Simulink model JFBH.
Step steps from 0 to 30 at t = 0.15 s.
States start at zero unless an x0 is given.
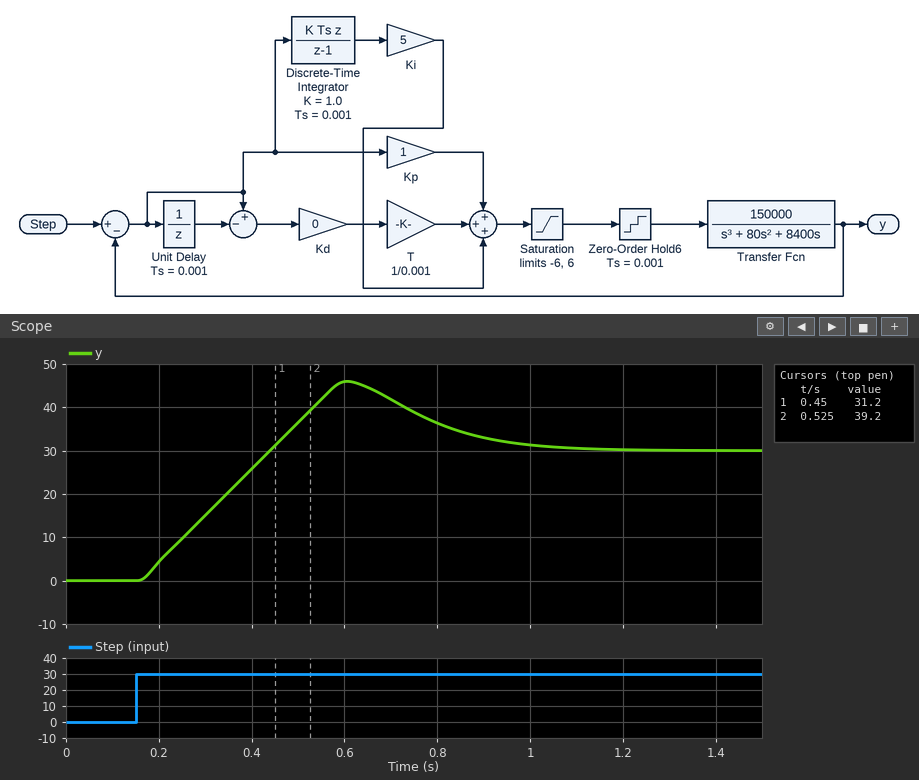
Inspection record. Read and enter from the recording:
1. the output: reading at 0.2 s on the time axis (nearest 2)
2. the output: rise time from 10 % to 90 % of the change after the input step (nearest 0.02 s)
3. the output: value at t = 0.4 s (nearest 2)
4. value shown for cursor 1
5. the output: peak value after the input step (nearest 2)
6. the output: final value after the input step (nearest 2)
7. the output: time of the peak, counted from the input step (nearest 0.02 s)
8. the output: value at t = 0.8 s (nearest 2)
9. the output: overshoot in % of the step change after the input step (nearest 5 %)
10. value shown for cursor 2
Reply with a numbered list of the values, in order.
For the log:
1. 4
2. 0.22 s
3. 26
4. 31.2
5. 46
6. 30
7. 0.46 s
8. 36
9. 55 %
10. 39.2
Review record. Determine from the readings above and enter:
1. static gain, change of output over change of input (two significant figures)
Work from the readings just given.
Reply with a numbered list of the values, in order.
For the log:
1. 1.0
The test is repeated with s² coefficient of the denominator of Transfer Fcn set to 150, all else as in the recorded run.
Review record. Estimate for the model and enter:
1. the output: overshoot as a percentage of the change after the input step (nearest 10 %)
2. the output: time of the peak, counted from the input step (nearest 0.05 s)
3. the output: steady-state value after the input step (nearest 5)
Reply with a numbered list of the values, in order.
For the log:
1. 60 %
2. 0.50 s
3. 30
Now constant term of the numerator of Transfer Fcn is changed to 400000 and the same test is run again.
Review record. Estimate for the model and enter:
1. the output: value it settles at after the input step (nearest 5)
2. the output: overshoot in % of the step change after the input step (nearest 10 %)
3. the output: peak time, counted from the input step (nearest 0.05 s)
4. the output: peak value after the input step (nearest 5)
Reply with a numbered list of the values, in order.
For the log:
1. 30
2. 30 %
3. 0.15 s
4. 40
